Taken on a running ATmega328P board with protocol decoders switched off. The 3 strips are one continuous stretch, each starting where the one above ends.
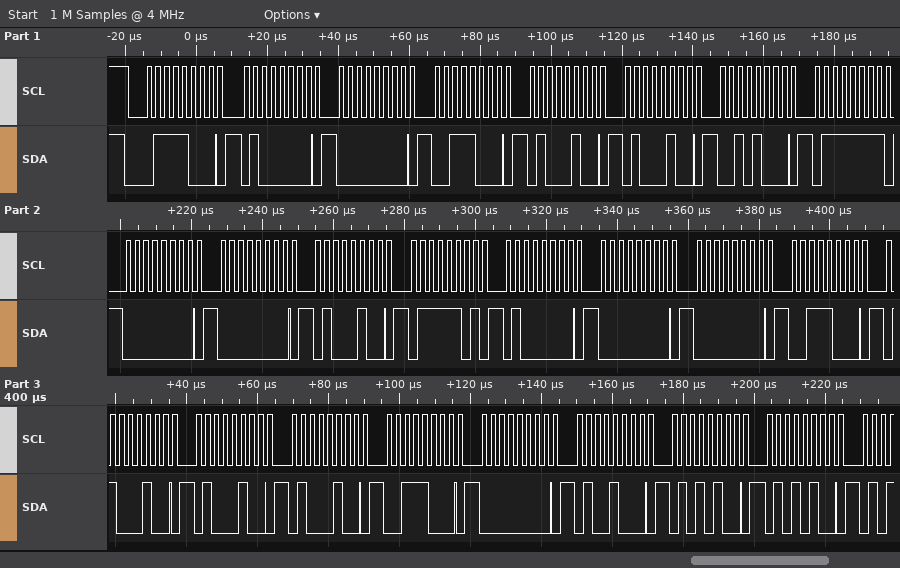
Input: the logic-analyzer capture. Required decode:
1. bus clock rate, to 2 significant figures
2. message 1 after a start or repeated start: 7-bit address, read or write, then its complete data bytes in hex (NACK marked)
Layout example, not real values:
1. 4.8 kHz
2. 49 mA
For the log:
1. 400 kHz
2. 0x3C write: 40 00 38 44 44 28 7F 00 00 44 7D 40 00 00 38 44 44 44 38 00 48 54 54
